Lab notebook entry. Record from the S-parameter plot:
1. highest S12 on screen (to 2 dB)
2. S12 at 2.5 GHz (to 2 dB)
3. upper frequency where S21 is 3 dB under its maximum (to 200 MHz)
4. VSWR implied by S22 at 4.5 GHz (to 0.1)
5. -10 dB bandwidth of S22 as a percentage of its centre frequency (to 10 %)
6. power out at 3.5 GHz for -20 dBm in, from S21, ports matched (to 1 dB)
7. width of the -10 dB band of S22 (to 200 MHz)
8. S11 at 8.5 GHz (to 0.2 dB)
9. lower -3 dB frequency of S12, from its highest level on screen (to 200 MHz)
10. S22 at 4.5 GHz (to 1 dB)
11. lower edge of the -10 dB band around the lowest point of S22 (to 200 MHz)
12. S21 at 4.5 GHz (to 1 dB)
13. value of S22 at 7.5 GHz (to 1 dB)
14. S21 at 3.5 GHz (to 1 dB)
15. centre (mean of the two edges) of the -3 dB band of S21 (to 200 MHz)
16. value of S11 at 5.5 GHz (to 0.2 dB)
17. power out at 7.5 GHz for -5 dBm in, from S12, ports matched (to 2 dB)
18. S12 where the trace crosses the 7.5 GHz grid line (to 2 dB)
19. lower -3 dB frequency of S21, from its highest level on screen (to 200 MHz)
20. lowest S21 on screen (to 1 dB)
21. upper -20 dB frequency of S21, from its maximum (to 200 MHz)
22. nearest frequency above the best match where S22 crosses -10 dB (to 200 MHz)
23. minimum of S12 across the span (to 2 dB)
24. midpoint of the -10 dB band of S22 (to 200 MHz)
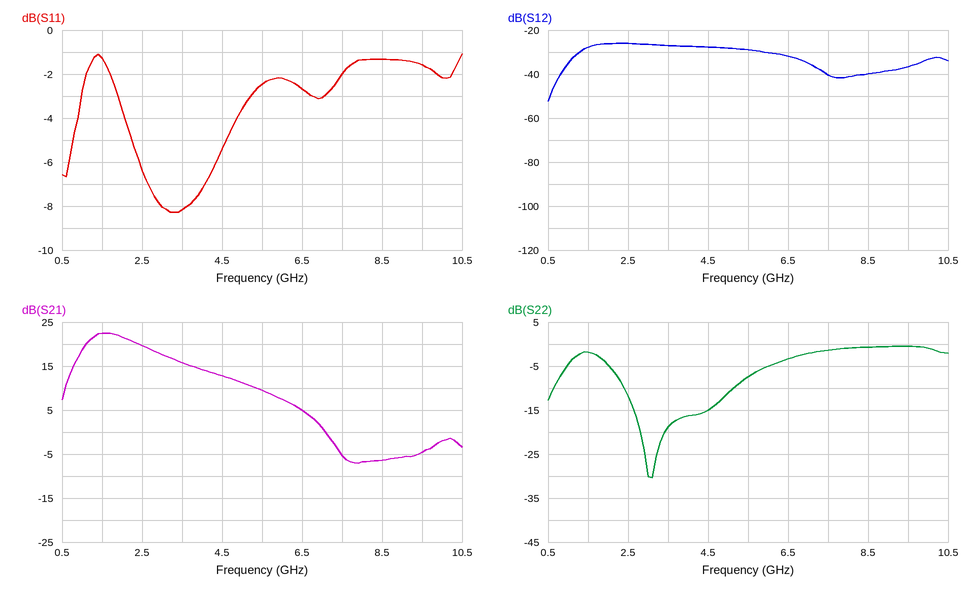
-26 dB
-26 dB
2.6 GHz
1.4
70 %
-4 dBm
2.8 GHz
-1.4 dB
1.4 GHz
-15 dB
2.4 GHz
13 dB
-1 dB
16 dB
1.8 GHz
-2.4 dB
-46 dBm
-40 dB
1.0 GHz
-7 dB
6.8 GHz
5.2 GHz
-52 dB
3.8 GHz
